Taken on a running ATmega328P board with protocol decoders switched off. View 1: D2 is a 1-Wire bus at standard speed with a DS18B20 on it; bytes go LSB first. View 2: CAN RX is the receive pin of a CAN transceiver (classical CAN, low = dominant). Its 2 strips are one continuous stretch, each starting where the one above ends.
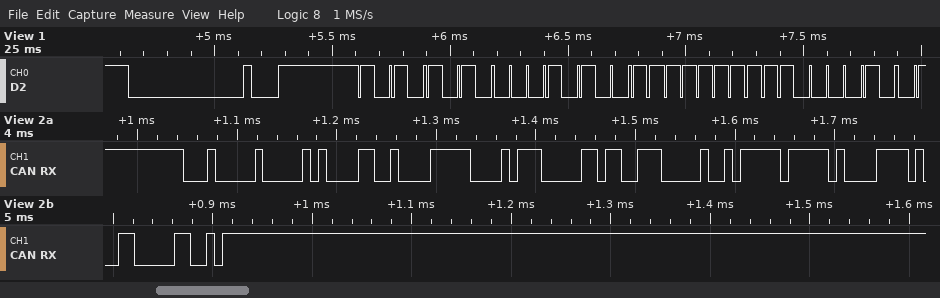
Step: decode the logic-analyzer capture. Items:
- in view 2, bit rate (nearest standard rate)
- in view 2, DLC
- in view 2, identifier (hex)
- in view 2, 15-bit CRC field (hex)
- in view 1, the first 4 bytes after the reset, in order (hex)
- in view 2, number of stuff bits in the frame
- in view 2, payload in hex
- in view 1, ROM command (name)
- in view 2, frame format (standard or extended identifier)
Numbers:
125 kbit/s
8
0x100
0x5304
55 28 FF 43
8
64 3E 2E 0B 38 0B FF 87
Match ROM
standard
